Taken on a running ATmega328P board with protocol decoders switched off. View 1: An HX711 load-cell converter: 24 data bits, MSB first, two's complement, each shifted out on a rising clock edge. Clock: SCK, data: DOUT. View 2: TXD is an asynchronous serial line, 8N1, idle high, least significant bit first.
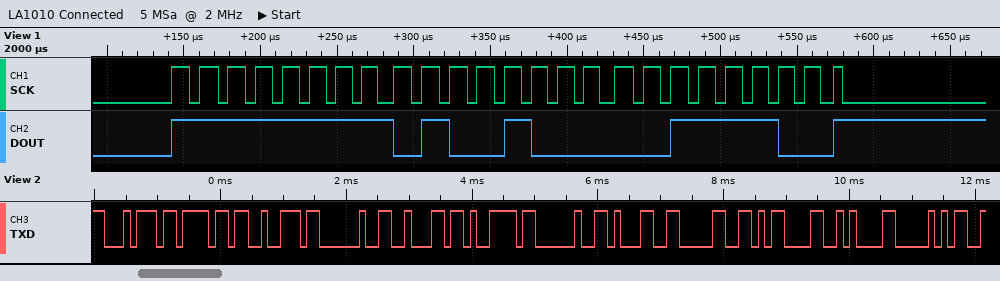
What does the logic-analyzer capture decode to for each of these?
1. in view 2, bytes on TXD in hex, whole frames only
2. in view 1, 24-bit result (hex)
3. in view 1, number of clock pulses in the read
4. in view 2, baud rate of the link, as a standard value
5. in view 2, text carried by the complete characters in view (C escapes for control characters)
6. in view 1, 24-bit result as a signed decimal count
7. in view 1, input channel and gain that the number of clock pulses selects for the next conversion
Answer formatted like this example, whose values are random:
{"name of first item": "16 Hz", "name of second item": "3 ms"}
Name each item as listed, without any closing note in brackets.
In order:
{"in view 2, bytes on TXD in hex, whole frames only": "74 6F 72 20 62 79 20 31 30 0D 0A 50", "in view 1, 24-bit result": "0xFF483C", "in view 1, number of clock pulses in the read": "25", "in view 2, baud rate of the link, as a standard value": "9600 baud", "in view 2, text carried by the complete characters in view": "\"tor by 10\\r\\nP\"", "in view 1, 24-bit result as a signed decimal count": "-47044", "in view 1, input channel and gain that the number of clock pulses selects for the next conversion": "channel A, gain 128"}
